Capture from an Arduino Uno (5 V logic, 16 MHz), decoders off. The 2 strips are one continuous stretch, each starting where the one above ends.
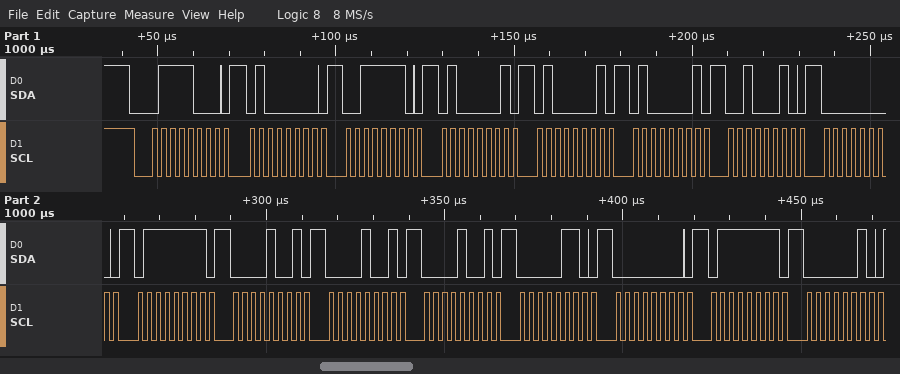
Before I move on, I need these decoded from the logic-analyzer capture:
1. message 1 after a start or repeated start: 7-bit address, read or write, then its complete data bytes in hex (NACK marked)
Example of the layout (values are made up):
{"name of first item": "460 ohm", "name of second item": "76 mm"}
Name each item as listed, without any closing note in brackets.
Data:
{"message 1 after a start or repeated start: 7-bit address, read or write, then its complete data bytes in hex": "0x3C write: 40 3E 41 41 41 22 00 7F 09 09 09 06 00 7F 02"}
